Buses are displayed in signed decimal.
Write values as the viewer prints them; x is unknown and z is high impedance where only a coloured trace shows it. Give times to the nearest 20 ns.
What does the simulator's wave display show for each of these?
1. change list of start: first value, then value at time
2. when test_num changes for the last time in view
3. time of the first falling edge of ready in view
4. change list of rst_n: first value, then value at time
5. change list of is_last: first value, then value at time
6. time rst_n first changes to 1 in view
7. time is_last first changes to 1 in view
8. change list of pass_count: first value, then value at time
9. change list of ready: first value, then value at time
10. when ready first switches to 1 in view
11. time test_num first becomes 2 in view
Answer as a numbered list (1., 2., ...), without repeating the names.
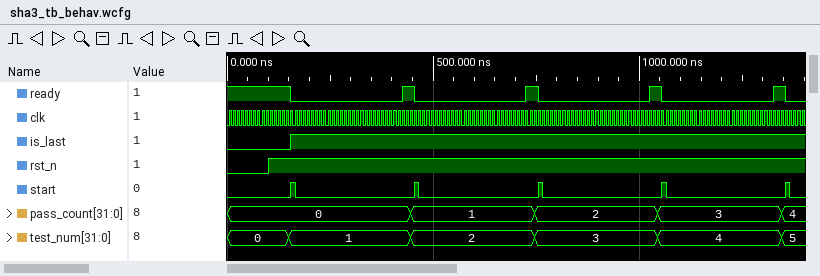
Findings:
1. 0, 1 at 160 ns, 0 at 160 ns, 1 at 460 ns, 0 at 460 ns, 1 at 760 ns, 0 at 760 ns, 1 at 1060 ns, 0 at 1060 ns, 1 at 1360 ns, 0 at 1360 ns
2. 1340 ns
3. 160 ns
4. 0, 1 at 100 ns
5. 0, 1 at 160 ns
6. 100 ns
7. 160 ns
8. 0, 1 at 440 ns, 2 at 740 ns, 3 at 1040 ns, 4 at 1340 ns
9. 1, 0 at 160 ns, 1 at 420 ns, 0 at 460 ns, 1 at 720 ns, 0 at 760 ns, 1 at 1020 ns, 0 at 1060 ns, 1 at 1320 ns, 0 at 1360 ns
10. 420 ns
11. 440 ns
